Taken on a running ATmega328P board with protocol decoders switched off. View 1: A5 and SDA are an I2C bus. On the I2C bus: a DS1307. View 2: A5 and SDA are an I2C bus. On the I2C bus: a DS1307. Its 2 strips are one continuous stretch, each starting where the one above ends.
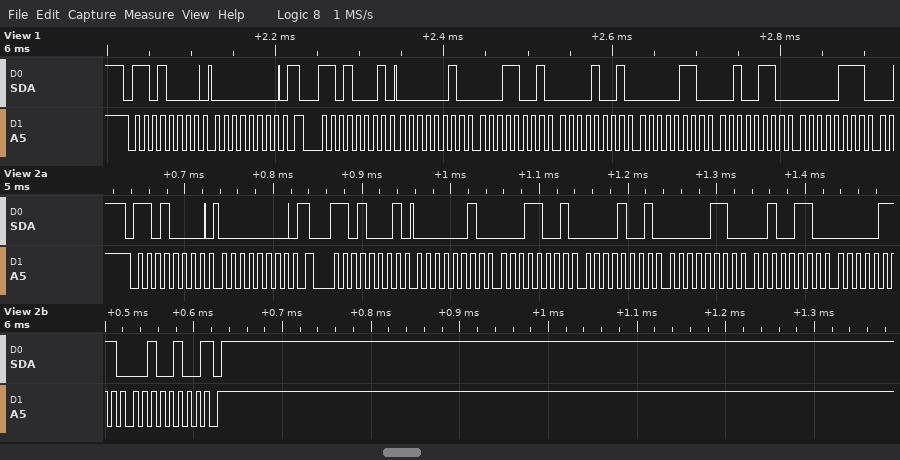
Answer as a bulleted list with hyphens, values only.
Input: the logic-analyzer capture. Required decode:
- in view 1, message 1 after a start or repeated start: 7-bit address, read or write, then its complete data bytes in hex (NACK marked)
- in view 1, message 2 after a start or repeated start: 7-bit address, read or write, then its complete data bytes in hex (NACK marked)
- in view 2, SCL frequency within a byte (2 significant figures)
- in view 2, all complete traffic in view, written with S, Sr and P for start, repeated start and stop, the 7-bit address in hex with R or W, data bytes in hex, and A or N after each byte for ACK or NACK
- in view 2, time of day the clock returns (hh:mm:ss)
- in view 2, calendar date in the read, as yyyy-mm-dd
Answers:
- 0x68 write: 00
- 0x68 read: 02 19 09 06 26 07
- 100 kHz
- S 68W A 00 A Sr 68R A 02 A 19 A 09 A 06 A 26 A 07 A 24 N P
- 09:19:02
- 2024-07-26
